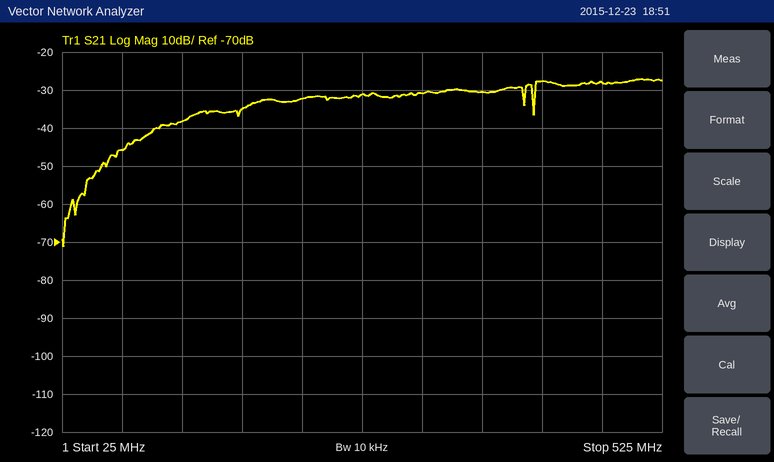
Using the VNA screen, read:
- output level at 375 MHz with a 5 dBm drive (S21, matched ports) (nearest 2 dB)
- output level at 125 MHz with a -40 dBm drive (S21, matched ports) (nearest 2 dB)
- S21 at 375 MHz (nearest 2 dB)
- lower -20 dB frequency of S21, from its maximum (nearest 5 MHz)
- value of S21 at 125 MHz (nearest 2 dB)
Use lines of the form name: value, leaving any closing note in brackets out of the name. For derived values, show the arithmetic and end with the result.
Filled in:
output level at 375 MHz with a 5 dBm drive (S21, matched ports): 5 dBm + (-30 dB) = -26 dBm
output level at 125 MHz with a -40 dBm drive (S21, matched ports): -40 dBm + (-38 dB) = -78 dBm
S21 at 375 MHz: -30 dB
lower -20 dB frequency of S21, from its maximum: 70 MHz
value of S21 at 125 MHz: -38 dB
